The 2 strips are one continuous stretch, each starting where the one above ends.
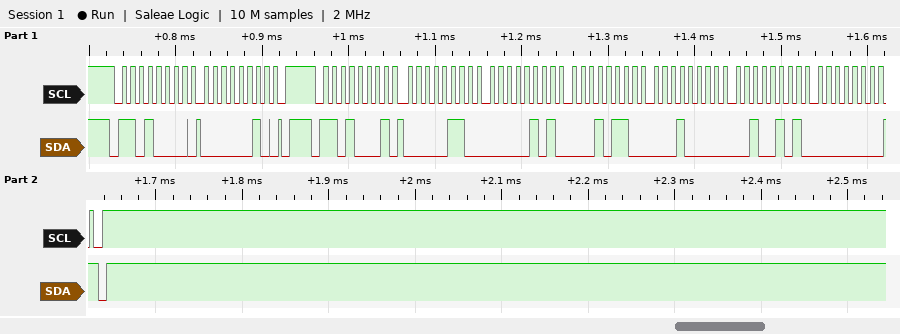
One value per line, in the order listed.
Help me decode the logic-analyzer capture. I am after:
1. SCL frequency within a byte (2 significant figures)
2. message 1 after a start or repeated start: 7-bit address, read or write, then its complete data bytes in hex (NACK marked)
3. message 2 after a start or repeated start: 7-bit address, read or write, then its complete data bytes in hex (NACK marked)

100 kHz
0x68 write: 02
0x68 read: 06 05 16 10 25 00 NACK
